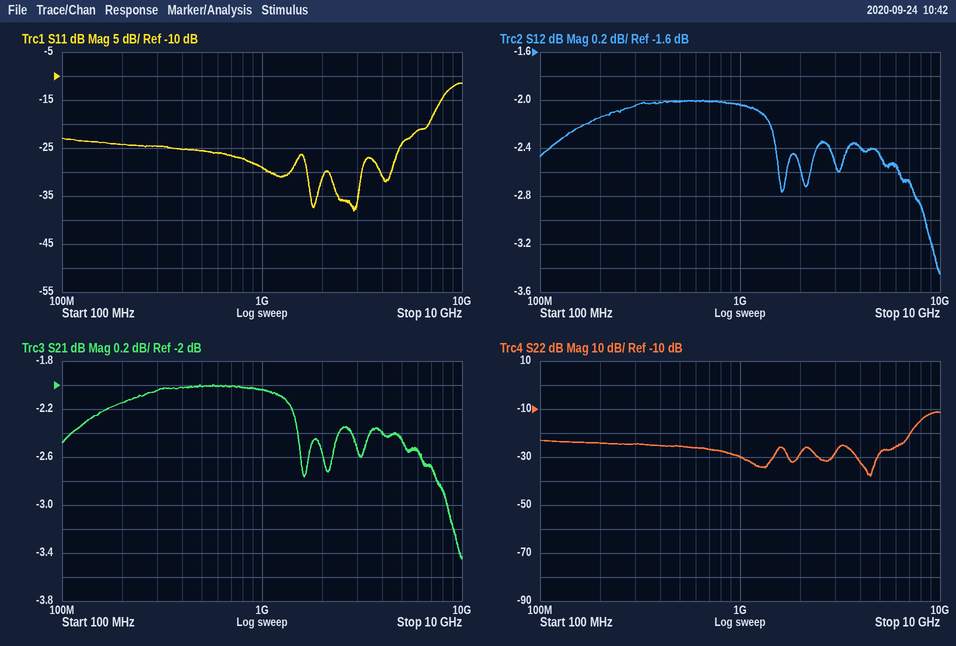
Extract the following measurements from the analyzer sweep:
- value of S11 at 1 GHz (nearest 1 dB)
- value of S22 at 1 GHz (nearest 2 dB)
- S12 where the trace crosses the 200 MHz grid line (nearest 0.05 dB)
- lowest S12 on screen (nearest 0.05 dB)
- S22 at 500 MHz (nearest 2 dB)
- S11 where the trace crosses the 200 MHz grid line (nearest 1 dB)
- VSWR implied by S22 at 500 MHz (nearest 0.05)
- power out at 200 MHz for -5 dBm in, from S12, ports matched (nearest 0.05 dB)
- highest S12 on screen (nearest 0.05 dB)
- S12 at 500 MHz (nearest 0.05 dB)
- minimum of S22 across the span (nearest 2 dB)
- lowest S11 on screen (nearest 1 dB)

-29 dB
-30 dB
-2.15 dB
-3.45 dB
-26 dB
-24 dB
1.10
-7.15 dBm
-2.00 dB
-2.00 dB
-38 dB
-38 dB
